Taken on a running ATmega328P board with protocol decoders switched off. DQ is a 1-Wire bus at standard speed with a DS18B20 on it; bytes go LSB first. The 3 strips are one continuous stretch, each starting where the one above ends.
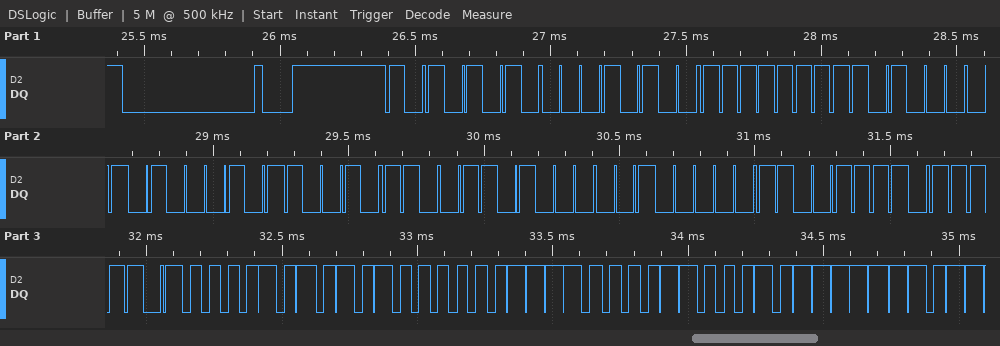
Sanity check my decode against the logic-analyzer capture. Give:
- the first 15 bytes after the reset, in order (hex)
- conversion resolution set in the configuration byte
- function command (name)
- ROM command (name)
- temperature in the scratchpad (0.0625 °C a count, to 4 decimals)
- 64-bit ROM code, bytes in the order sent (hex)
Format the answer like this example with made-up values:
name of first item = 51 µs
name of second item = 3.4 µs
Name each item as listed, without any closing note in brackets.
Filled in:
the first 15 bytes after the reset, in order = 55 28 FF 85 A2 69 16 04 F3 BE 50 05 1E 46 7F
conversion resolution set in the configuration byte = 12 bits
function command = Read Scratchpad
ROM command = Match ROM
temperature in the scratchpad = 85.0000 °C
64-bit ROM code, bytes in the order sent = 28 FF 85 A2 69 16 04 F3
